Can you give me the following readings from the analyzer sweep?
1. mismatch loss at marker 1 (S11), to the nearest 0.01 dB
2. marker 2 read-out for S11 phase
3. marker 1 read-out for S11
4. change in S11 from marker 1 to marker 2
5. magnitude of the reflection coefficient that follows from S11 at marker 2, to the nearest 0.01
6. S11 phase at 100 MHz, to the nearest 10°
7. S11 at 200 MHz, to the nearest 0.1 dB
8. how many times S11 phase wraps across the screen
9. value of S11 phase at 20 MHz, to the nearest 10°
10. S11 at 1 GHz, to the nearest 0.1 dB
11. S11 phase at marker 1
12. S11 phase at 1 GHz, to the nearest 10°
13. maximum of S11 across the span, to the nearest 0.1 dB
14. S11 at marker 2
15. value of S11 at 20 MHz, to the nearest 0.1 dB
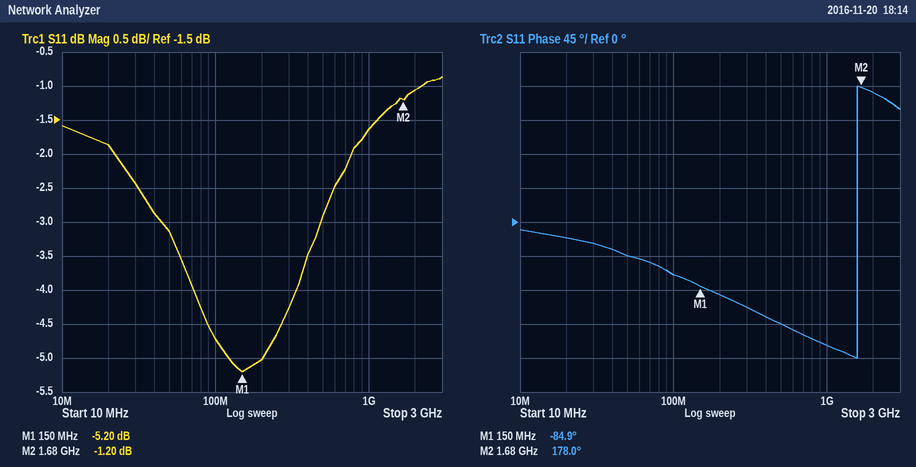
1.56 dB
178.0°
-5.20 dB
4.00 dB
0.87
-70°
-5.0 dB
1
-20°
-1.6 dB
-84.9°
-160°
-0.9 dB
-1.20 dB
-1.9 dB
